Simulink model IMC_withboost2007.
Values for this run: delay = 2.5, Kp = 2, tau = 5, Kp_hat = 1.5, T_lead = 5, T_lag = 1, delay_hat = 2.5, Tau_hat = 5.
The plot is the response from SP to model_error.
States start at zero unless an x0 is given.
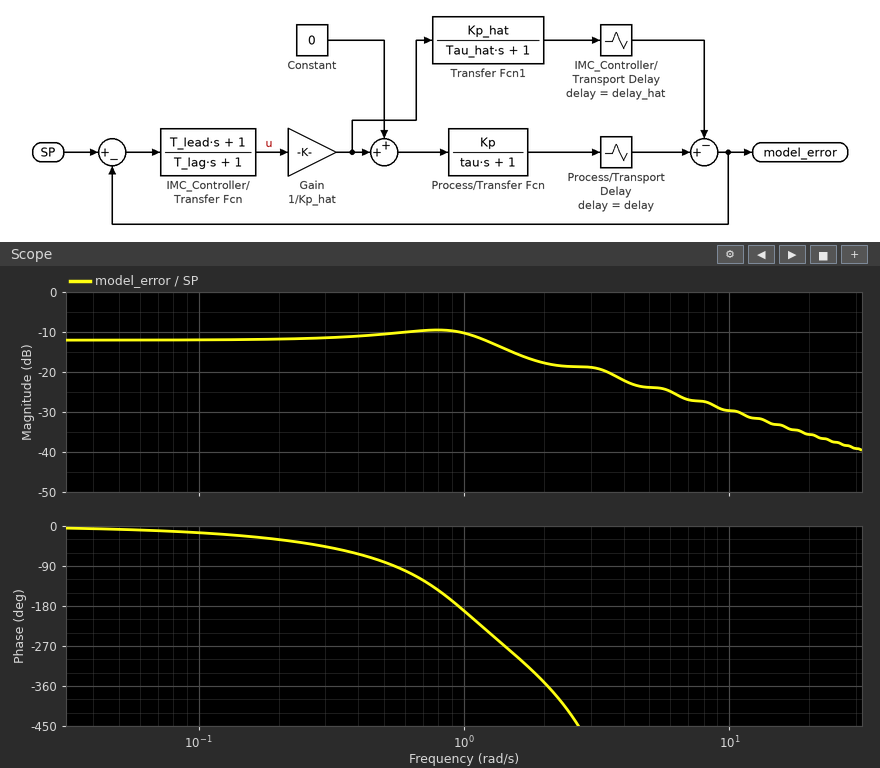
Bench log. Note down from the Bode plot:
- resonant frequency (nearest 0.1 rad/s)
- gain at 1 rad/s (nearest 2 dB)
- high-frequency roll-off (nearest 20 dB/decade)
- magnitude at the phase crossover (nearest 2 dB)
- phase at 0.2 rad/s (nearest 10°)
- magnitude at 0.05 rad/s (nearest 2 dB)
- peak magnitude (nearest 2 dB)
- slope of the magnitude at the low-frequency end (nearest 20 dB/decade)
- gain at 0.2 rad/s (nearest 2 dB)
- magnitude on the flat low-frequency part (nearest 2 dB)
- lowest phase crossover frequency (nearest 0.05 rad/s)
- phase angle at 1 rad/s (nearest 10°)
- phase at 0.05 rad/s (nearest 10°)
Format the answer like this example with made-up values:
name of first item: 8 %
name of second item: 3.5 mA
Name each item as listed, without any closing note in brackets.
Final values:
resonant frequency: 0.8 rad/s
gain at 1 rad/s: -10 dB
high-frequency roll-off: -20 dB/decade
magnitude at the phase crossover: -10 dB
phase at 0.2 rad/s: -30°
magnitude at 0.05 rad/s: -12 dB
peak magnitude: -10 dB
slope of the magnitude at the low-frequency end: 0 dB/decade
gain at 0.2 rad/s: -12 dB
magnitude on the flat low-frequency part: -12 dB
lowest phase crossover frequency: 0.95 rad/s
phase angle at 1 rad/s: -190°
phase at 0.05 rad/s: -10°
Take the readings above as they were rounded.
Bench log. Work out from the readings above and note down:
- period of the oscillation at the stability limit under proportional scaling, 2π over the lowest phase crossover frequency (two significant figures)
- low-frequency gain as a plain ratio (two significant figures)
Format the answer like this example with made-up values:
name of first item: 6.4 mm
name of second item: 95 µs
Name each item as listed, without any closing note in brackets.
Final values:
period of the oscillation at the stability limit under proportional scaling, 2π over the lowest phase crossover frequency: 6.6 s
low-frequency gain as a plain ratio: 0.25
